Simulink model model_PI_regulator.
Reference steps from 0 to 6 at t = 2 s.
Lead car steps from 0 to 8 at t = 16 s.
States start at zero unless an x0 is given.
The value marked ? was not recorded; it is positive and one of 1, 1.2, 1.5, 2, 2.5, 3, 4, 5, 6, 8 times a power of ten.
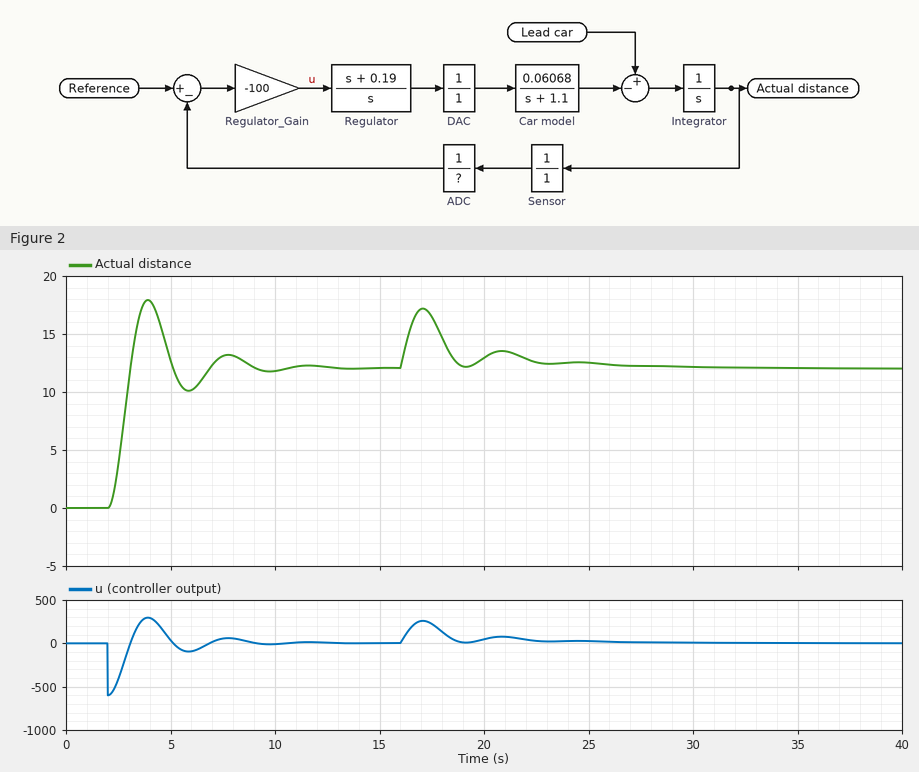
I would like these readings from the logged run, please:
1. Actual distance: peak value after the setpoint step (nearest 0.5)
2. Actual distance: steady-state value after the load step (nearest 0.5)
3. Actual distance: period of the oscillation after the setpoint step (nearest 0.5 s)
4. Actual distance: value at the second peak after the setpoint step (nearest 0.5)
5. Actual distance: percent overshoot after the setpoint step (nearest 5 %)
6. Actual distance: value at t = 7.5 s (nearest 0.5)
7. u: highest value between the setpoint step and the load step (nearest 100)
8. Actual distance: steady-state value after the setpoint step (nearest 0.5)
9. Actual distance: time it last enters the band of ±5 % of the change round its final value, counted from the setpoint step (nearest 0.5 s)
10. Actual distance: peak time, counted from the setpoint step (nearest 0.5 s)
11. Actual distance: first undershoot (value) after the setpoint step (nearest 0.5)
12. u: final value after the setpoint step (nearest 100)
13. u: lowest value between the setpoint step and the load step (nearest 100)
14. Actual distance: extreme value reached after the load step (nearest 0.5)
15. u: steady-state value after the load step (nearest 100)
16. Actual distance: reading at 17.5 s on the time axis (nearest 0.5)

18.0
12.0
4.0 s
13.0
50 %
13.0
300
12.0
6.5 s
2.0 s
10.0
0
-600
17.0
0
16.5
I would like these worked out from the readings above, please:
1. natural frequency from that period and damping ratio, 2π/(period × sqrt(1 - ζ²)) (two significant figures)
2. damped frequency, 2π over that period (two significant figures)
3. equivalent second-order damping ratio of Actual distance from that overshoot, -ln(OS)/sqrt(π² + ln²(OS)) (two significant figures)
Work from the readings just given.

1.6 rad/s
1.6 rad/s
0.22
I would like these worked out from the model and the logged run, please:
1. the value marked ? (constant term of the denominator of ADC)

2
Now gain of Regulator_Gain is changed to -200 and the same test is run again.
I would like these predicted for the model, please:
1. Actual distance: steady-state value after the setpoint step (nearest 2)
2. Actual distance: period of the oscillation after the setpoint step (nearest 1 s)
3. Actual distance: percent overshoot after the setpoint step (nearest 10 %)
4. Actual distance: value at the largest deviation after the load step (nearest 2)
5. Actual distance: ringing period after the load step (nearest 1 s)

12
3 s
60 %
16
3 s
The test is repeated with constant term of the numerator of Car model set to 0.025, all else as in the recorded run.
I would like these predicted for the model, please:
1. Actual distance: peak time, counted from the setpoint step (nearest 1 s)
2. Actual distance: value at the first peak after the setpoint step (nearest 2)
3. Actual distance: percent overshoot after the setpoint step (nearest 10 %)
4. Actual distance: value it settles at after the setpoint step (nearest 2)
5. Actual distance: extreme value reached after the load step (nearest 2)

3 s
16
40 %
12
20
